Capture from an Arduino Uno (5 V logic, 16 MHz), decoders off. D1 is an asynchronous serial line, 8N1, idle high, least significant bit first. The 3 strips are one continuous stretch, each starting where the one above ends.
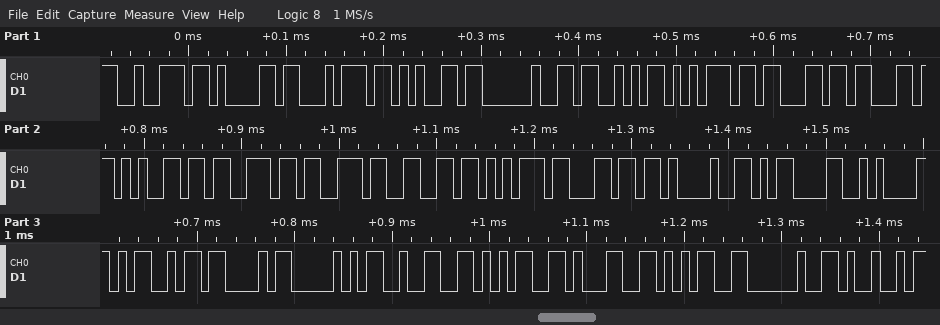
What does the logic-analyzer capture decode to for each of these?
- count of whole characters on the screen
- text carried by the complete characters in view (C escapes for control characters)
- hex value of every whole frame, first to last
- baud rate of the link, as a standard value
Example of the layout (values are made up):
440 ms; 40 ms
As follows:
27; "rate Successful!\r\nMCP2515 I"; 72 61 74 65 20 53 75 63 63 65 73 73 66 75 6C 21 0D 0A 4D 43 50 32 35 31 35 20 49; 115200 baud
